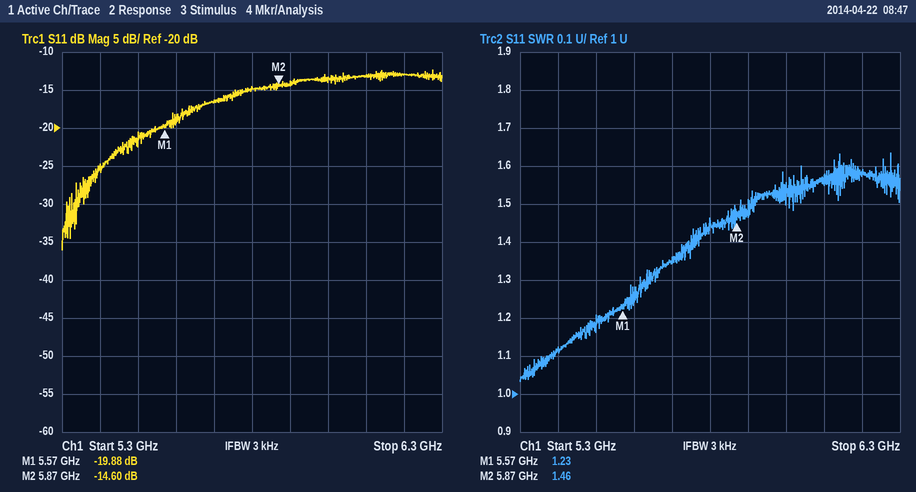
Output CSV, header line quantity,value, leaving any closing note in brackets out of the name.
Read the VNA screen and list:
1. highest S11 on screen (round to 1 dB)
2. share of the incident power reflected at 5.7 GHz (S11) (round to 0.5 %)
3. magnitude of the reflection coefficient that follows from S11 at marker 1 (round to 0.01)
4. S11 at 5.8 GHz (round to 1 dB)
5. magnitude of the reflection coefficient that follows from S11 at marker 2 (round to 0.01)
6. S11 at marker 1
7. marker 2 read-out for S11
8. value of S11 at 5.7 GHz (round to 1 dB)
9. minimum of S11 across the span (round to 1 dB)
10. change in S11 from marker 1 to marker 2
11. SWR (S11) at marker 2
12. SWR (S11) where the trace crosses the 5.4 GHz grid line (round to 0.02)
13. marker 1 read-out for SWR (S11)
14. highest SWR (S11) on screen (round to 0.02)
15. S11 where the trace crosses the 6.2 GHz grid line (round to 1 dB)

quantity,value
highest S11 on screen,-12 dB
share of the incident power reflected at 5.7 GHz (S11),2.0 %
magnitude of the reflection coefficient that follows from S11 at marker 1,0.10
S11 at 5.8 GHz,-15 dB
magnitude of the reflection coefficient that follows from S11 at marker 2,0.19
S11 at marker 1,-19.88 dB
marker 2 read-out for S11,-14.60 dB
value of S11 at 5.7 GHz,-17 dB
minimum of S11 across the span,-36 dB
change in S11 from marker 1 to marker 2,5.28 dB
SWR (S11) at marker 2,1.46
SWR (S11) where the trace crosses the 5.4 GHz grid line,1.12
marker 1 read-out for SWR,1.23
highest SWR (S11) on screen,1.64
S11 where the trace crosses the 6.2 GHz grid line,-13 dB
